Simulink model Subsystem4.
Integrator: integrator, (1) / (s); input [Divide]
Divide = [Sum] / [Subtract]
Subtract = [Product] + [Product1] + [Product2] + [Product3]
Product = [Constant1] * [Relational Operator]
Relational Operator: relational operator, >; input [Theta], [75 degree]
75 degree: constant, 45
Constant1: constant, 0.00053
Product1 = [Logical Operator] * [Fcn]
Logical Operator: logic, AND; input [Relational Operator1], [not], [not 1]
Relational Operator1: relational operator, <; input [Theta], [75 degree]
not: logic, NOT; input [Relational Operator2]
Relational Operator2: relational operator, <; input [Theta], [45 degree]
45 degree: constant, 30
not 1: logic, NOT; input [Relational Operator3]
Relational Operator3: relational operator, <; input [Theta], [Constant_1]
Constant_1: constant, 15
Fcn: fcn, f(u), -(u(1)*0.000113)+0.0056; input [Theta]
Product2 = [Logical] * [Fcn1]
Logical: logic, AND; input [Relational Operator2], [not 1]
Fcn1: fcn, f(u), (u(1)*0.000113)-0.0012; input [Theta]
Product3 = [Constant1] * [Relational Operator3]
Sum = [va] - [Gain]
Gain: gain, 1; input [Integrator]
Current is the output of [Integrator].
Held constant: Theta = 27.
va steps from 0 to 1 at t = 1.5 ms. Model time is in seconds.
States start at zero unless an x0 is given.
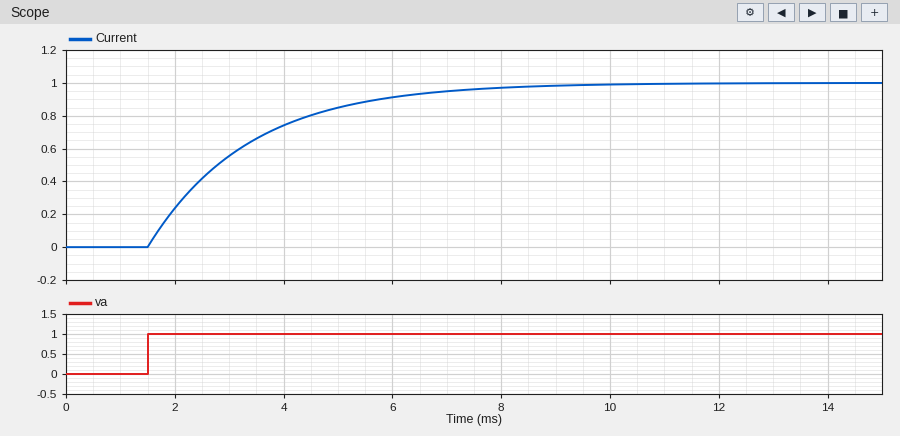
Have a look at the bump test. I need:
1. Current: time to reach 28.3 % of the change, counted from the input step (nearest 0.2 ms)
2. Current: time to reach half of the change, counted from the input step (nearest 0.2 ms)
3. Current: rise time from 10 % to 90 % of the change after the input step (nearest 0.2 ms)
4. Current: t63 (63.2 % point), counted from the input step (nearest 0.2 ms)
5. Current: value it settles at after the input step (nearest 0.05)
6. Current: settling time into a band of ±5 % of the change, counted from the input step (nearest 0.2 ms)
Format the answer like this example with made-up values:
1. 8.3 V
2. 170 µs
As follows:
1. 0.6 ms
2. 1.2 ms
3. 4.0 ms
4. 1.8 ms
5. 1.00
6. 5.6 ms
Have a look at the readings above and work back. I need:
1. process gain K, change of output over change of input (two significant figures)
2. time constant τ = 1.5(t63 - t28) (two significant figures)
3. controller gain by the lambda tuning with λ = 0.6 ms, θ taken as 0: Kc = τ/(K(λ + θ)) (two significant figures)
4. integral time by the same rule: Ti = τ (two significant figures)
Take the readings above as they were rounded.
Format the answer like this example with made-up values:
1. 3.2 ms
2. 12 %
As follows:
1. 1.0
2. 1.8 ms
3. 3.0
4. 1.8 ms
